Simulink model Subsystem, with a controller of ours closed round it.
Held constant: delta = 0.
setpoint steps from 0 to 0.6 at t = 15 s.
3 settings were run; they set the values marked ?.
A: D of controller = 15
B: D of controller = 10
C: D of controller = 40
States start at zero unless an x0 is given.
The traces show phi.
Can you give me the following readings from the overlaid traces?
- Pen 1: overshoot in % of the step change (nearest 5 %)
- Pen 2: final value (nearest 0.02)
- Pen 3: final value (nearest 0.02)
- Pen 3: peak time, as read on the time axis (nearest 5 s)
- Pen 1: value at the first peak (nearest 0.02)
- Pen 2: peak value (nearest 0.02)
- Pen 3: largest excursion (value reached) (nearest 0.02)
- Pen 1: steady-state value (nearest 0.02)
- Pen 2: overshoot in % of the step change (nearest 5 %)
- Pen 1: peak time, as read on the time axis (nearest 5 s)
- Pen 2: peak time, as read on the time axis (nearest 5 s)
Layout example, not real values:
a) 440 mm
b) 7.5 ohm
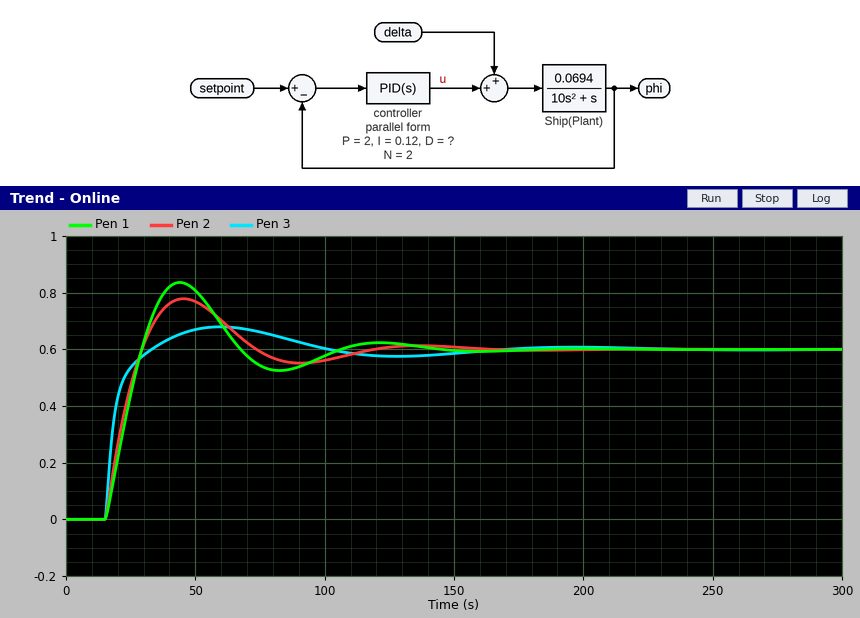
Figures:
a) 40 %
b) 0.60
c) 0.60
d) 60 s
e) 0.84
f) 0.78
g) 0.68
h) 0.60
i) 30 %
j) 45 s
k) 45 s
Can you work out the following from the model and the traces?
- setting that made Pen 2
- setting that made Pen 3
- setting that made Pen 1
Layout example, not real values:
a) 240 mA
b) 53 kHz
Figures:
a) A
b) C
c) B
